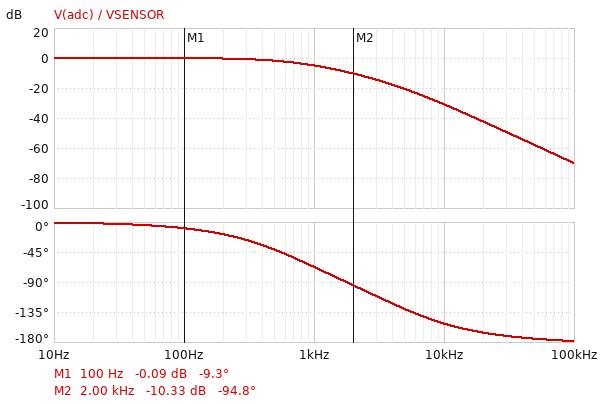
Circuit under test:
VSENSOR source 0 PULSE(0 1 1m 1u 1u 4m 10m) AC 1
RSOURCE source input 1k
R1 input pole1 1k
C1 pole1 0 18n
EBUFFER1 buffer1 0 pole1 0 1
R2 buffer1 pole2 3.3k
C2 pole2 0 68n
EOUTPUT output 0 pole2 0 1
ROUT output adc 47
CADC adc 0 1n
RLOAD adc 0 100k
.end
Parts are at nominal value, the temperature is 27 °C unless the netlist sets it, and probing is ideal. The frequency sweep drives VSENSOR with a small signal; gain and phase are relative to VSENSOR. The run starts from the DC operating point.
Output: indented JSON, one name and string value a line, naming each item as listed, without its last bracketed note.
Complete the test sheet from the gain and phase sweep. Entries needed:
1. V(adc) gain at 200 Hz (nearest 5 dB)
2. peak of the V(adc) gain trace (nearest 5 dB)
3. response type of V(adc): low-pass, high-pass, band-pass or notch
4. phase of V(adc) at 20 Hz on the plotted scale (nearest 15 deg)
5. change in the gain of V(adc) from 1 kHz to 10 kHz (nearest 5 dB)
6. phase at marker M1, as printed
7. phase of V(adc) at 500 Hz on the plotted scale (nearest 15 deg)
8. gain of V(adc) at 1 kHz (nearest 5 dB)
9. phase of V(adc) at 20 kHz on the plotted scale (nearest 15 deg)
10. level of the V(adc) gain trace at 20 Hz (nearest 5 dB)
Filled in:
{
  "V(adc) gain at 200 Hz": "0 dB",
  "peak of the V(adc) gain trace": "0 dB",
  "response type of V(adc): low-pass, high-pass, band-pass or notch": "low-pass",
  "phase of V(adc) at 20 Hz on the plotted scale": "0 deg",
  "change in the gain of V(adc) from 1 kHz to 10 kHz": "-25 dB",
  "phase at marker M1, as printed": "-9.3 deg",
  "phase of V(adc) at 500 Hz on the plotted scale": "-45 deg",
  "gain of V(adc) at 1 kHz": "-5 dB",
  "phase of V(adc) at 20 kHz on the plotted scale": "-165 deg",
  "level of the V(adc) gain trace at 20 Hz": "0 dB"
}
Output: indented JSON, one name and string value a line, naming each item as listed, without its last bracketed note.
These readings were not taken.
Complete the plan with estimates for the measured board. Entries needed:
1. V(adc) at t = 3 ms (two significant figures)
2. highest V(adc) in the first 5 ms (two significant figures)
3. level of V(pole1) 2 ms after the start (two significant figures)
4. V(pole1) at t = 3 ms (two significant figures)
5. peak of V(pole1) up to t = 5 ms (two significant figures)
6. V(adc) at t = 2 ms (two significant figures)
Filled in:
{
  "V(adc) at t = 3 ms": "1.0 V",
  "highest V(adc) in the first 5 ms": "1.0 V",
  "level of V(pole1) 2 ms after the start": "1.0 V",
  "V(pole1) at t = 3 ms": "1.0 V",
  "peak of V(pole1) up to t = 5 ms": "1.0 V",
  "V(adc) at t = 2 ms": "990 mV"
}
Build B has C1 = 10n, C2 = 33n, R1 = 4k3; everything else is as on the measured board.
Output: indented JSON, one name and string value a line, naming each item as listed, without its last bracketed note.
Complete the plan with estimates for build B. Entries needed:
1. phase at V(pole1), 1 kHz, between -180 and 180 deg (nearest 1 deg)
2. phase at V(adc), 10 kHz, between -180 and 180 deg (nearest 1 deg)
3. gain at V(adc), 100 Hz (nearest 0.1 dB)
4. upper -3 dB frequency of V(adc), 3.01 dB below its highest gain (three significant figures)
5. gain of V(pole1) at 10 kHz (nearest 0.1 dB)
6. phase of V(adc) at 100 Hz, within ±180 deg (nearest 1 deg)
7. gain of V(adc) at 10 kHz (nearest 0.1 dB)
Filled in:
{
  "phase at V(pole1), 1 kHz, between -180 and 180 deg": "-18 deg",
  "phase at V(adc), 10 kHz, between -180 and 180 deg": "-155 deg",
  "gain at V(adc), 100 Hz": "0 dB",
  "upper -3 dB frequency of V(adc), 3.01 dB below its highest gain": "1.23 kHz",
  "gain of V(pole1) at 10 kHz": "-10.8 dB",
  "phase of V(adc) at 100 Hz, within ±180 deg": "-6 deg",
  "gain of V(adc) at 10 kHz": "-27.6 dB"
}
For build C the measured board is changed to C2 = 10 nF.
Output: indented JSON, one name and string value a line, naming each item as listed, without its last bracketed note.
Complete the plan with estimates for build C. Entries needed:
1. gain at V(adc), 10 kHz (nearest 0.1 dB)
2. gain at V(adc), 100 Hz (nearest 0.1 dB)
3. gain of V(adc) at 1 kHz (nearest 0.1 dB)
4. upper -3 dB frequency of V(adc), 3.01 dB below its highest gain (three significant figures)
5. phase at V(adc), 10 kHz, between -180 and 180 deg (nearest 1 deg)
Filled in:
{
  "gain at V(adc), 10 kHz": "-15.1 dB",
  "gain at V(adc), 100 Hz": "0 dB",
  "gain of V(adc) at 1 kHz": "-0.4 dB",
  "upper -3 dB frequency of V(adc), 3.01 dB below its highest gain": "2.97 kHz",
  "phase at V(adc), 10 kHz, between -180 and 180 deg": "-131 deg"
}
